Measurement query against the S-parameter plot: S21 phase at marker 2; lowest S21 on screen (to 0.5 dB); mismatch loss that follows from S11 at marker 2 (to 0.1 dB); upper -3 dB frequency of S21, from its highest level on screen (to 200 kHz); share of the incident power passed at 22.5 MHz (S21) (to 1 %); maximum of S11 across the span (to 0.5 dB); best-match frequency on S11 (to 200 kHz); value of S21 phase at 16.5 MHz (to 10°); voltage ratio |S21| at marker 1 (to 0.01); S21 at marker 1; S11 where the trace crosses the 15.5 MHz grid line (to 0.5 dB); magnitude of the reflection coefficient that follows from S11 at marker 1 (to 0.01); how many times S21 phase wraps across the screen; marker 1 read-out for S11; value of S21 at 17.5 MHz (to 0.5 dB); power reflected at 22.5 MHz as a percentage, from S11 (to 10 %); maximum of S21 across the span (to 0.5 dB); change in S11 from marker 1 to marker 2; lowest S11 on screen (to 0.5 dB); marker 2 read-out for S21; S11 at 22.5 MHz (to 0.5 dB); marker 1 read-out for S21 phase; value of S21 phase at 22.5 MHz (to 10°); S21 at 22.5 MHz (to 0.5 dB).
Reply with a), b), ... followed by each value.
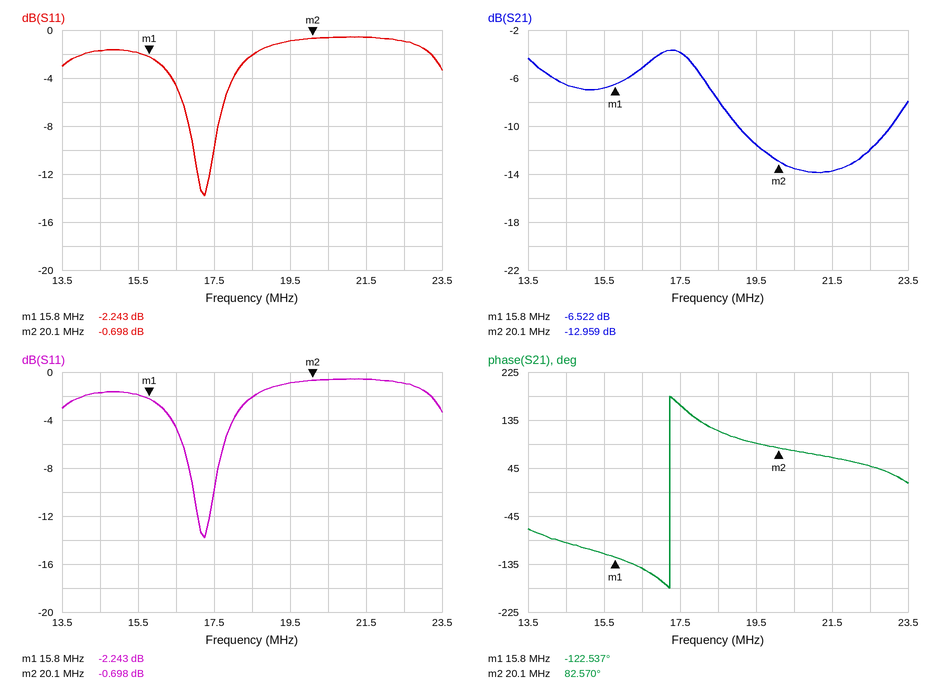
a) 82.570°
b) -14.0 dB
c) 8.3 dB
d) 18.2 MHz
e) 6 %
f) -0.5 dB
g) 17.2 MHz
h) -140°
i) 0.47
j) -6.522 dB
k) -2.0 dB
l) 0.77
m) 1
n) -2.243 dB
o) -4.0 dB
p) 80 %
q) -3.5 dB
r) 1.545 dB
s) -14.0 dB
t) -12.959 dB
u) -1.0 dB
v) -122.537°
w) 50°
x) -12.0 dB
